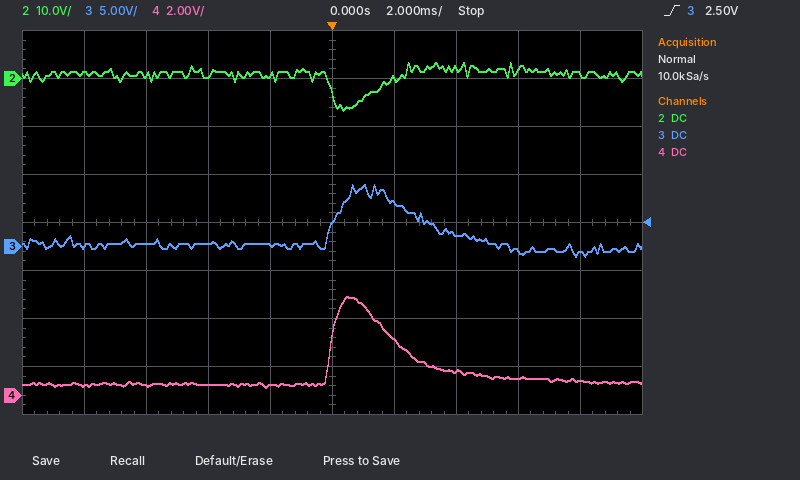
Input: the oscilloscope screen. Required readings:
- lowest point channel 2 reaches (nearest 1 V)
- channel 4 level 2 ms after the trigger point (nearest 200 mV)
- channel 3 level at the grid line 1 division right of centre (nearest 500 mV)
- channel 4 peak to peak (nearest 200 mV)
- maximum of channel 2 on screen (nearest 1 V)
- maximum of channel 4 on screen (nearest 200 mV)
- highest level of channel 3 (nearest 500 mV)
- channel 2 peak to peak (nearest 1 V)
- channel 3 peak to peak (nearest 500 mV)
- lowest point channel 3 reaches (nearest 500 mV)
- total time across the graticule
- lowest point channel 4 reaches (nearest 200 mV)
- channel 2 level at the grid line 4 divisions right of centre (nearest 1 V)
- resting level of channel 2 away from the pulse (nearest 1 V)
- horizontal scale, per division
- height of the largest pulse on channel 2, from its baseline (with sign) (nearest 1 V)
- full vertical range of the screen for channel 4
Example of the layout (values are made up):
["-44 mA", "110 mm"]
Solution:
["-7 V", "2.4 V", "4.5 V", "3.8 V", "3 V", "4.2 V", "6.5 V", "10 V", "7.5 V", "-1.0 V", "20 ms", "400 mV", "1 V", "1 V", "2 ms", "-8 V", "16 V"]
